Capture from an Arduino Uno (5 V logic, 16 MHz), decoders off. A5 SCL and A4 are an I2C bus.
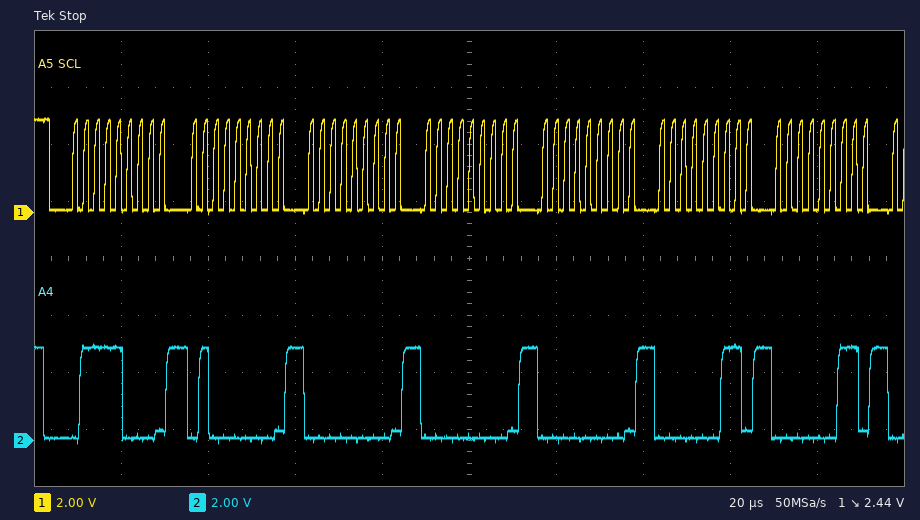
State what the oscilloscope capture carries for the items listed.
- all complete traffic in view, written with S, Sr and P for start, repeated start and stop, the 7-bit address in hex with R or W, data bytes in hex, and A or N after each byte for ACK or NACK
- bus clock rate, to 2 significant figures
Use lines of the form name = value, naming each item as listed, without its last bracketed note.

all complete traffic in view, written with S, Sr and P for start, repeated start and stop, the 7-bit address in hex with R or W, data bytes in hex, and A or N after each byte for ACK or NACK = S 3CW A 40 A 00 A 00 A 00 A 03 A 03 A
bus clock rate, to 2 significant figures = 400 kHz
